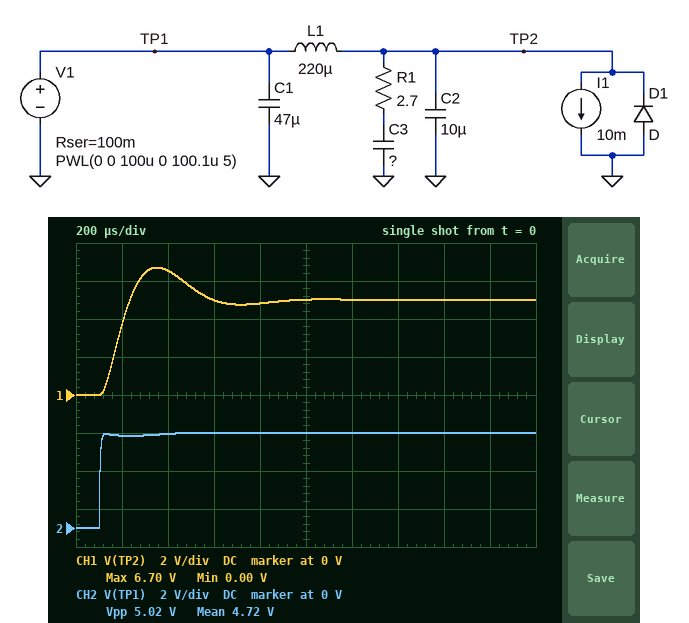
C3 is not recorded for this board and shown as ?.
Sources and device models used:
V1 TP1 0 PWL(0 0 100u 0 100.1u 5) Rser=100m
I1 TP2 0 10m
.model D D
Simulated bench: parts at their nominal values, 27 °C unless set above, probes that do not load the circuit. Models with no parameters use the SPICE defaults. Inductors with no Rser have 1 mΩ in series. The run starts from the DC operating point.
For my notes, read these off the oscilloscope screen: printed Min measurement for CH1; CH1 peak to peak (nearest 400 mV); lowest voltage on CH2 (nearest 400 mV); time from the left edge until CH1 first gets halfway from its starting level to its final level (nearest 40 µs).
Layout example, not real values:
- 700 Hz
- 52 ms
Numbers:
- 0.00 V
- 6.8 V
- 0 V
- 160 µs
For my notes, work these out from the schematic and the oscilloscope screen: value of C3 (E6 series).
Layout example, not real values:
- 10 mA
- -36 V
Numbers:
- 47 µF
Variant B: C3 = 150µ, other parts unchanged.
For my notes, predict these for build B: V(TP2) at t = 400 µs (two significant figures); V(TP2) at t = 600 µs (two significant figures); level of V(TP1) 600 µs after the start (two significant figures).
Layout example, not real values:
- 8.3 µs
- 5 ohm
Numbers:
- 5.6 V
- 5.4 V
- 4.9 V
